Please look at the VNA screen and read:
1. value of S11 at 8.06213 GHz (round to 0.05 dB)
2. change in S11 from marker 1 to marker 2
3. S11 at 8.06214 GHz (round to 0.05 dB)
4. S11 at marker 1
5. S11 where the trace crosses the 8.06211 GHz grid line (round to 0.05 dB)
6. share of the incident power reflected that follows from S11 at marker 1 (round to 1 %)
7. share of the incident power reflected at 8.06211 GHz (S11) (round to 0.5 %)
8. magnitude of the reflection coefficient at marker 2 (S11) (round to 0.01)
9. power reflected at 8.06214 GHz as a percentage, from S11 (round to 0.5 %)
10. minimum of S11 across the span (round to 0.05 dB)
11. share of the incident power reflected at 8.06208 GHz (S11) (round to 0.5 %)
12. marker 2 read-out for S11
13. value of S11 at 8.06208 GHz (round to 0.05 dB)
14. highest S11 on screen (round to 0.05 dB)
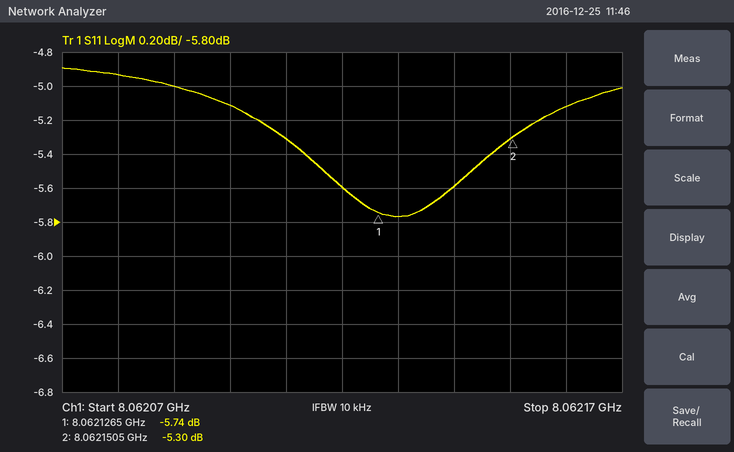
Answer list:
-5.75 dB
0.44 dB
-5.60 dB
-5.74 dB
-5.30 dB
27 %
29.5 %
0.54
27.5 %
-5.75 dB
32.0 %
-5.30 dB
-4.95 dB
-4.90 dB
